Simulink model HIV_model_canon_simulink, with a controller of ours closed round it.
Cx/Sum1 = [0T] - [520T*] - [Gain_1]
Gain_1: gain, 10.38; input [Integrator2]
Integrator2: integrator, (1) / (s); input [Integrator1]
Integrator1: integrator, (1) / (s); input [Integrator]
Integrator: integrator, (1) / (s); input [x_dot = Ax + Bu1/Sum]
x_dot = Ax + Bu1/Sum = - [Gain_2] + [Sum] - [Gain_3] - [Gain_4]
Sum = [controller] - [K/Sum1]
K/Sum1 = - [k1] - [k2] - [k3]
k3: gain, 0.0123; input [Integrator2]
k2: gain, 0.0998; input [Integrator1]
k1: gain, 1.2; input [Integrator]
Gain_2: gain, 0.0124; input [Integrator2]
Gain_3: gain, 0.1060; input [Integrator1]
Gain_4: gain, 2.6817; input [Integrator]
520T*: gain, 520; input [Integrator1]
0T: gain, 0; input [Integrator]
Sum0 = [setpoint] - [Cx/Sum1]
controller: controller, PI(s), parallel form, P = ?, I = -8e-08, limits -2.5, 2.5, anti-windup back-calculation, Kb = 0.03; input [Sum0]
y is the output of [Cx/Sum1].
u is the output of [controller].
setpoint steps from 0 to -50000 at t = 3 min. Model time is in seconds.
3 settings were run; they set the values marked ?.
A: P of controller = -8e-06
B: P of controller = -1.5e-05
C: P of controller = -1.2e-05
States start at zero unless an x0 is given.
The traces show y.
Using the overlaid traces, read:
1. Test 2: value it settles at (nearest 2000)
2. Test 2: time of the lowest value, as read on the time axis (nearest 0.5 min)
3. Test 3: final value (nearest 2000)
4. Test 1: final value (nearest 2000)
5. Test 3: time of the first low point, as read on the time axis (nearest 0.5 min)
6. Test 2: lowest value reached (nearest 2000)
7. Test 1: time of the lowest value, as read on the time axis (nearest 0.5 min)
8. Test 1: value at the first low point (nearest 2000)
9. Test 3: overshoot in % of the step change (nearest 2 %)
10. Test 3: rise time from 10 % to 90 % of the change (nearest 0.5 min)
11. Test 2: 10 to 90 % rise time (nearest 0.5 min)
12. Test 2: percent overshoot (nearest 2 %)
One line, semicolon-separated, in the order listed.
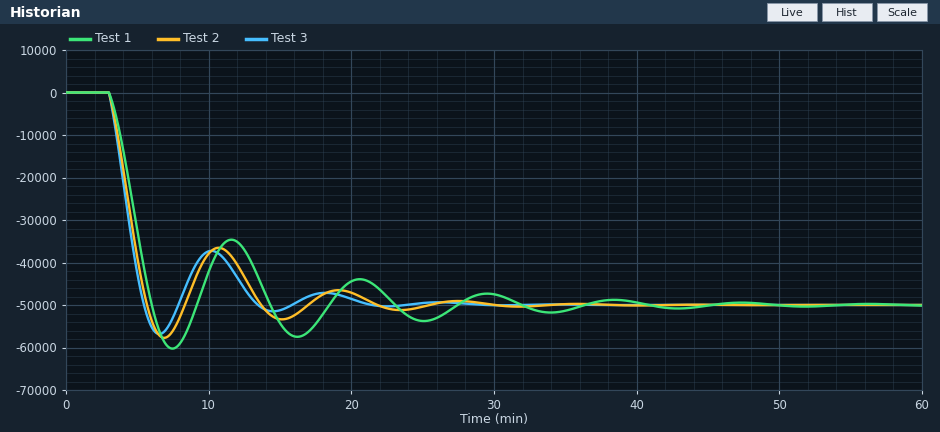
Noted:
-50000; 7.0 min; -50000; -50000; 6.5 min; -58000; 7.5 min; -60000; 14 %; 2.0 min; 2.0 min; 16 %
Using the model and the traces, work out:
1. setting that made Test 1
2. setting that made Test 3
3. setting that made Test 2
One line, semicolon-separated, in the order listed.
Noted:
A; B; C
